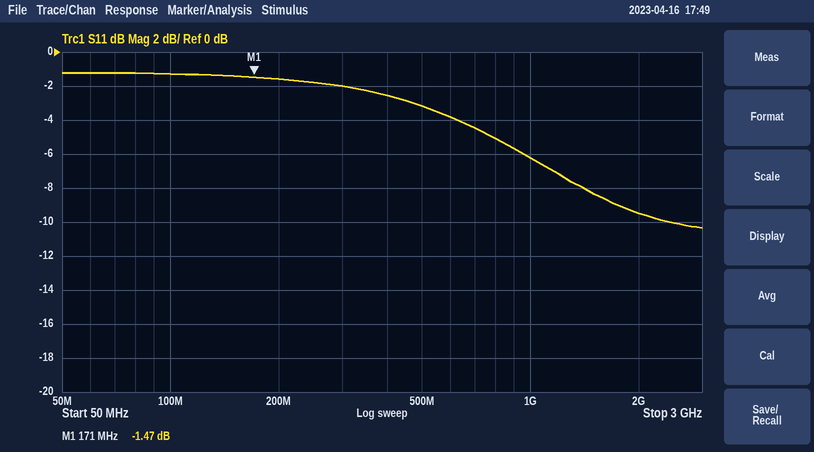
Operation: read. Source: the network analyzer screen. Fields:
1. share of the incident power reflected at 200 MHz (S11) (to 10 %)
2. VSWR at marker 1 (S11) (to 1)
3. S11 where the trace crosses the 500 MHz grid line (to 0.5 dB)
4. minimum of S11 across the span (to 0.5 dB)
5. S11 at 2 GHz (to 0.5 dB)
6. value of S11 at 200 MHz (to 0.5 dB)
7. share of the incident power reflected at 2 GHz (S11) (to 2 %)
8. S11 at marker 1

70 %
12
-3.0 dB
-10.5 dB
-9.5 dB
-1.5 dB
12 %
-1.47 dB
